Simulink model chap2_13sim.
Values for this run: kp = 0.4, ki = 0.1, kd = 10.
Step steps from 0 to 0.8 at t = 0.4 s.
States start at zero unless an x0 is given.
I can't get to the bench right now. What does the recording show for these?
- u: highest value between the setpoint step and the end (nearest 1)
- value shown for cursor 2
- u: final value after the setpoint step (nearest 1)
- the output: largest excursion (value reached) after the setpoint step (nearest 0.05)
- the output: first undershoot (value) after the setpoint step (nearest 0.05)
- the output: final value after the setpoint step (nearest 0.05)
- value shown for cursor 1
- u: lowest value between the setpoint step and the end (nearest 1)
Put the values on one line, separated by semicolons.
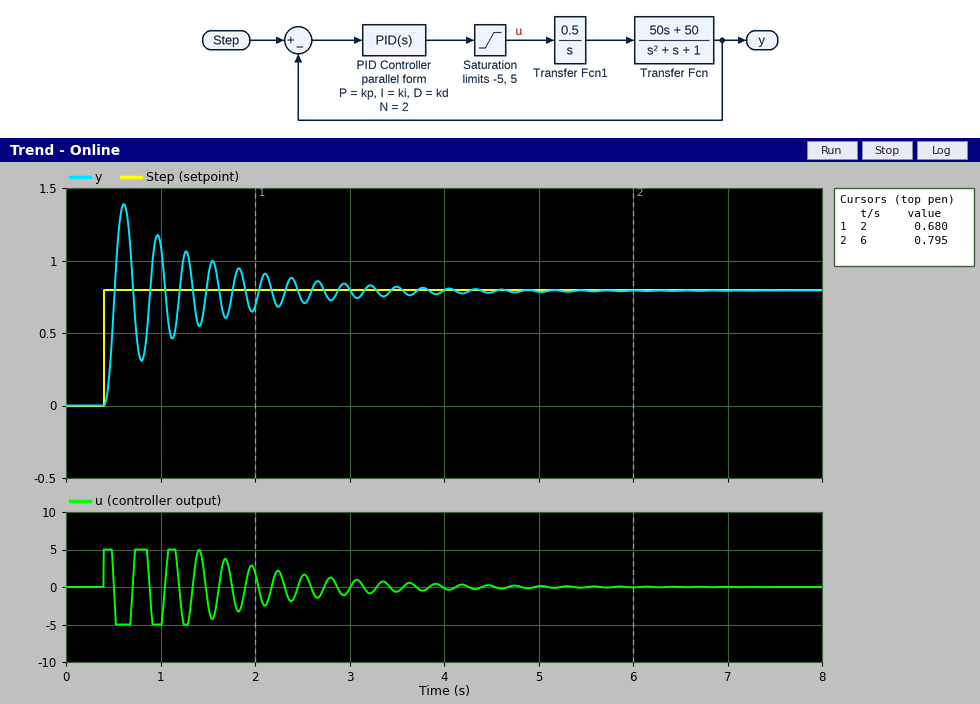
5; 0.795; 0; 1.40; 0.30; 0.80; 0.680; -5
